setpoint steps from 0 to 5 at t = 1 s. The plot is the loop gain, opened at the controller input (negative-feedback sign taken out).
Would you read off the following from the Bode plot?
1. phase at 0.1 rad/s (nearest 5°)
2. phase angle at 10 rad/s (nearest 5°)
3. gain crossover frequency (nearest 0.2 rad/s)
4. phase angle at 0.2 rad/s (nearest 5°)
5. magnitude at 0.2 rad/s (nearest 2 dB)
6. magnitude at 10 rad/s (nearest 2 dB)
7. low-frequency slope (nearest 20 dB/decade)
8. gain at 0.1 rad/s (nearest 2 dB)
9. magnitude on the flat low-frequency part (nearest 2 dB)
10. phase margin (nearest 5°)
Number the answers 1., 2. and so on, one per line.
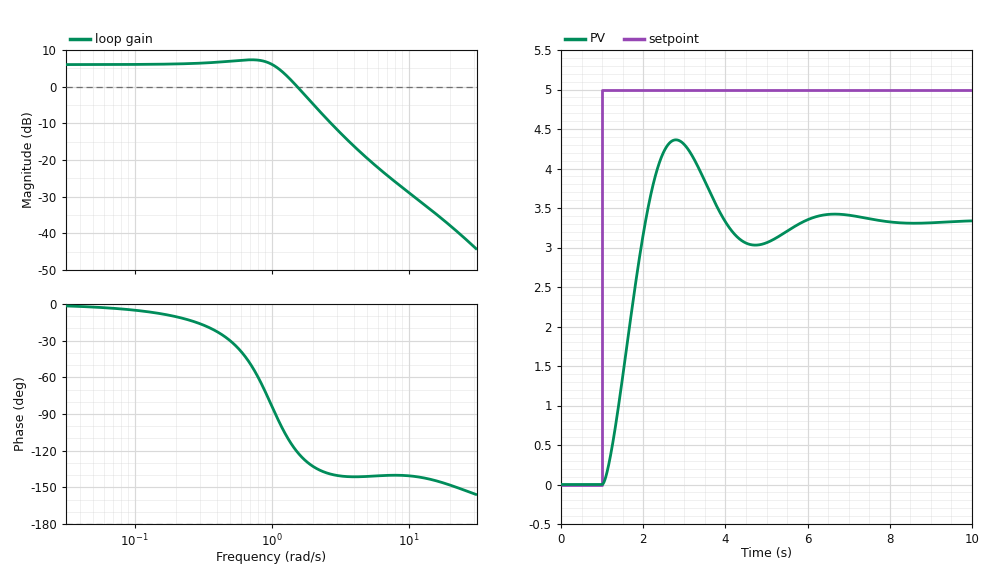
1. -5°
2. -140°
3. 1.6 rad/s
4. -10°
5. 6 dB
6. -28 dB
7. 0 dB/decade
8. 6 dB
9. 6 dB
10. 60°
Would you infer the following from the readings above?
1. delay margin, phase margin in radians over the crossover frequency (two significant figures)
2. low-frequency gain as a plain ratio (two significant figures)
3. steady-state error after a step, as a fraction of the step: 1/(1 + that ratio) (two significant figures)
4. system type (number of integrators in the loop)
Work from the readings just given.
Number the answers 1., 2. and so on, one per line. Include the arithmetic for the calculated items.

1. 60 × π / 180 / 1.6 = 0.65 s
2. 10^(6 / 20) = 2.0
3. 1 / (1 + 2) = 0.33
4. 0
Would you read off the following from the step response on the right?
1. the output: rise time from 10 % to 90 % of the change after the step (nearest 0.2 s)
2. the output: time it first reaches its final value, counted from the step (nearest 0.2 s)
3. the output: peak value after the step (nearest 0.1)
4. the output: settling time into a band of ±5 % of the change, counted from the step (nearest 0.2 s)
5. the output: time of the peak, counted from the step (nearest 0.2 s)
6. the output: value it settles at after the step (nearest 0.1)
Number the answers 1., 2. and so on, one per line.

1. 0.8 s
2. 1.0 s
3. 4.4
4. 4.4 s
5. 1.8 s
6. 3.3
